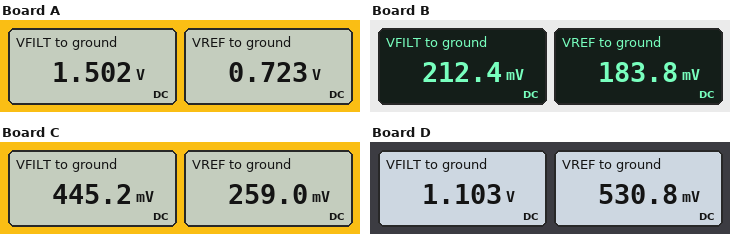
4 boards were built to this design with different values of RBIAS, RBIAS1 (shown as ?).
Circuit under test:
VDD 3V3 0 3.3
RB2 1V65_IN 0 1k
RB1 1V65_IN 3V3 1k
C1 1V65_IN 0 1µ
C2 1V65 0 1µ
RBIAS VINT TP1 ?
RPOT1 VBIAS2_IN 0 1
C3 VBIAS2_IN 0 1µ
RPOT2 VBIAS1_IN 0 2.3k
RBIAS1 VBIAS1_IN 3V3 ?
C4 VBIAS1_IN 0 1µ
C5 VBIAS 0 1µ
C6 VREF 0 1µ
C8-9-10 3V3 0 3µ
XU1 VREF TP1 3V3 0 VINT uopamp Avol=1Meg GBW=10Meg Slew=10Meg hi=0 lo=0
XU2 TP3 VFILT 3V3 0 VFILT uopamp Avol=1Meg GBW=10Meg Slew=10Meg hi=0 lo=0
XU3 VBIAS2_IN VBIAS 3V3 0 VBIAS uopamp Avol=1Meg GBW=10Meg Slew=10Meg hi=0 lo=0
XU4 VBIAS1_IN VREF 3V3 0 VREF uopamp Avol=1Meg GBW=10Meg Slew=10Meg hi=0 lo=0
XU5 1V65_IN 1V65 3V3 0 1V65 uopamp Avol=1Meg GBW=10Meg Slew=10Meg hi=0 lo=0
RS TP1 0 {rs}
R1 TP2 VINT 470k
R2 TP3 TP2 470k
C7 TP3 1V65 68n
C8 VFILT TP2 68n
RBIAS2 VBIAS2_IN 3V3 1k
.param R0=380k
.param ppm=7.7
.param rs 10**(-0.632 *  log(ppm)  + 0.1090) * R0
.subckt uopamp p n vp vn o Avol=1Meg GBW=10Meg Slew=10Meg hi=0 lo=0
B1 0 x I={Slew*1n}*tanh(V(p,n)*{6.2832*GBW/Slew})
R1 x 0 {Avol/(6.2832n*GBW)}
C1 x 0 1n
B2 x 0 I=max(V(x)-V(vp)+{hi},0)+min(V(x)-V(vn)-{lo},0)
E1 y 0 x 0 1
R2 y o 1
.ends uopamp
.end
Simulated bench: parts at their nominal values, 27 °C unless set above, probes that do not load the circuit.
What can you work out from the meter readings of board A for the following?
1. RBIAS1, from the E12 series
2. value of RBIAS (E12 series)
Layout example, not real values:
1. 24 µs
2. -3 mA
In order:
1. 8.2 kΩ
2. 27 kΩ
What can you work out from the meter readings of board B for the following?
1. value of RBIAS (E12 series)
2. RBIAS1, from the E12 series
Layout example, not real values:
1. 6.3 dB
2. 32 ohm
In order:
1. 3.9 kΩ
2. 39 kΩ
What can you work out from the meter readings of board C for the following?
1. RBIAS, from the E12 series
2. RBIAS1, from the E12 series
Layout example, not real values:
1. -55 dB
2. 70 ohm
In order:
1. 18 kΩ
2. 27 kΩ
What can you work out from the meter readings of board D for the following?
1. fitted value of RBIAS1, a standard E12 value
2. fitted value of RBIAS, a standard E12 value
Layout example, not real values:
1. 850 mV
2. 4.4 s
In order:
1. 12 kΩ
2. 27 kΩ
